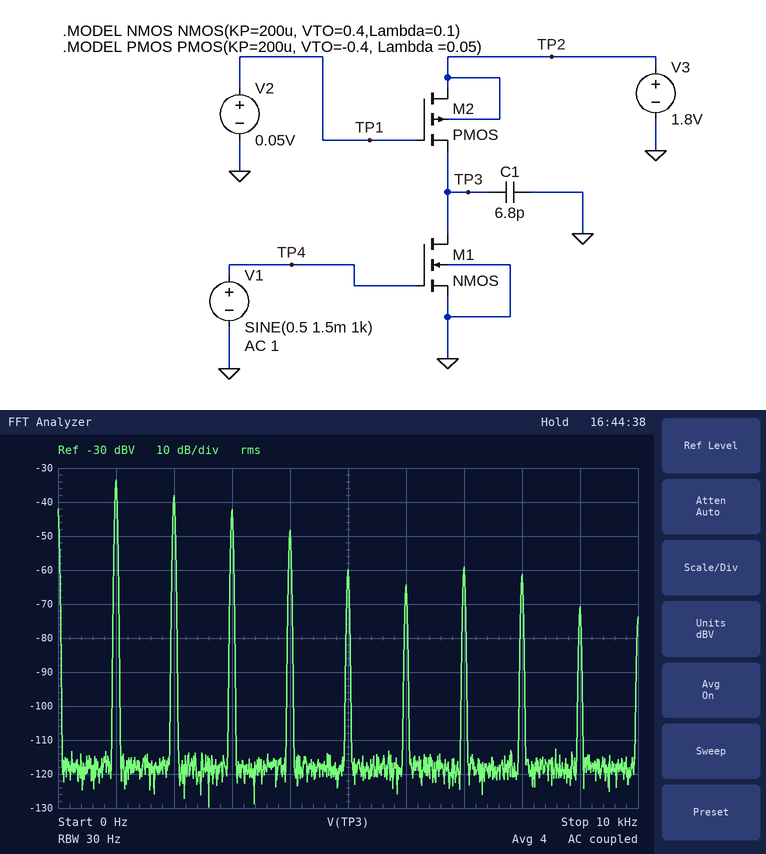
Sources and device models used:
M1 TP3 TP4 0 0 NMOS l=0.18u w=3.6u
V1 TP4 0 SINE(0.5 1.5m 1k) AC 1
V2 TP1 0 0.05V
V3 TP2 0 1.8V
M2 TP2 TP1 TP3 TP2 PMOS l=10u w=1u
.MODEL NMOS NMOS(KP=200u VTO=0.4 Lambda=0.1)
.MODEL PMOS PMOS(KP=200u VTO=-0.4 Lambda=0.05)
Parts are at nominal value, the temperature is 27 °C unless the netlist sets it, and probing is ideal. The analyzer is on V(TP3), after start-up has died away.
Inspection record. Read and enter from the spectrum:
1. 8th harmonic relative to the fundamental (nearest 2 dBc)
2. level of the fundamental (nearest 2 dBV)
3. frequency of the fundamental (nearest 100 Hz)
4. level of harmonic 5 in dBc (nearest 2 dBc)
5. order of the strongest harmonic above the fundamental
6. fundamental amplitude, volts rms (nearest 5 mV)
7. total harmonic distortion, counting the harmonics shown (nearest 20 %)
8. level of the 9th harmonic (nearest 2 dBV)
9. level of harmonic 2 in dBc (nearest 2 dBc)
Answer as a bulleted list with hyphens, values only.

- -28 dBc
- -34 dBV
- 1.0 kHz
- -26 dBc
- 2
- 20 mV
- 80 %
- -70 dBV
- -4 dBc
